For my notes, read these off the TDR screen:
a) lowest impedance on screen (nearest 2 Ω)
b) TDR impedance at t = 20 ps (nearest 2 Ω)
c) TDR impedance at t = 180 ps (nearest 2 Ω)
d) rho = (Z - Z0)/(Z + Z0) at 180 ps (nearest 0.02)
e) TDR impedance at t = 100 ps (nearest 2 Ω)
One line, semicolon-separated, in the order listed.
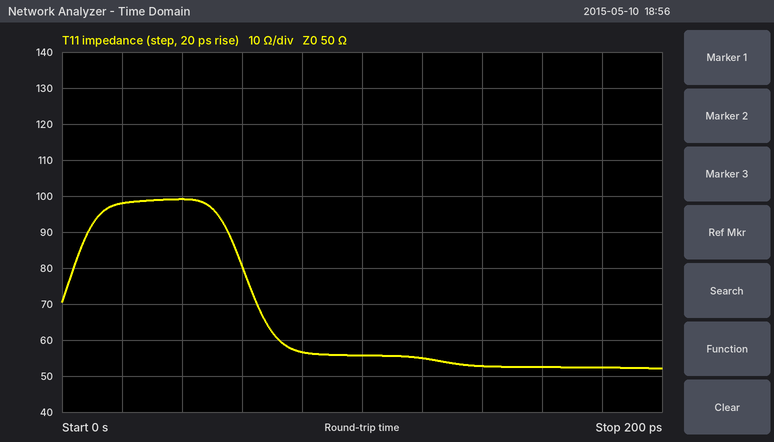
52 Ω; 98 Ω; 52 Ω; +0.02; 56 Ω
